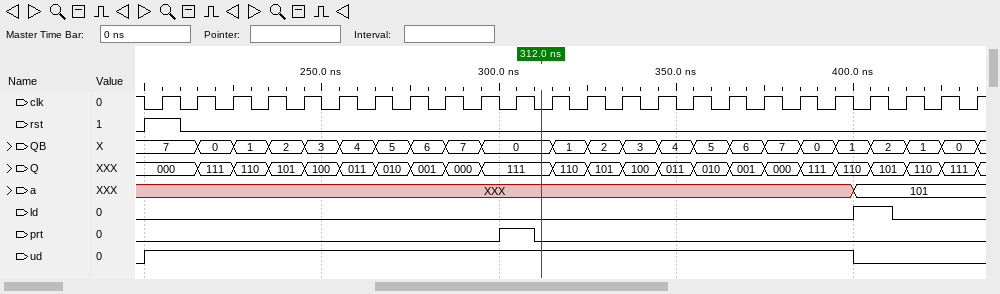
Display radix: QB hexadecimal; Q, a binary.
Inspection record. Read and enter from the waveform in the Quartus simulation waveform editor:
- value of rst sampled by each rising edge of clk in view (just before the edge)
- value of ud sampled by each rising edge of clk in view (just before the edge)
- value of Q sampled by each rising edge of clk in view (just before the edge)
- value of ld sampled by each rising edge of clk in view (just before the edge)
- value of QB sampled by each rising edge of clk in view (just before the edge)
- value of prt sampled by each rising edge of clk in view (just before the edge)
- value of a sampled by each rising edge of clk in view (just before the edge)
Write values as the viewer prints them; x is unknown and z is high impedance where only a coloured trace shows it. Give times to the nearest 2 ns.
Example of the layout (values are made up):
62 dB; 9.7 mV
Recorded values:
1 0 0 0 0 0 0 0 0 0 0 0 0 0 0 0 0 0 0 0 0 0 0 0; 1 1 1 1 1 1 1 1 1 1 1 1 1 1 1 1 1 1 1 1 0 0 0 0; 000, 000, 111, 110, 101, 100, 011, 010, 001, 000, 111, 111, 110, 101, 100, 011, 010, 001, 000, 111, 110, 101, 110, 111; 0 0 0 0 0 0 0 0 0 0 0 0 0 0 0 0 0 0 0 0 1 0 0 0; 7, 7, 0, 1, 2, 3, 4, 5, 6, 7, 0, 0, 1, 2, 3, 4, 5, 6, 7, 0, 1, 2, 1, 0; 0 0 0 0 0 0 0 0 0 0 1 0 0 0 0 0 0 0 0 0 0 0 0 0; XXX, XXX, XXX, XXX, XXX, XXX, XXX, XXX, XXX, XXX, XXX, XXX, XXX, XXX, XXX, XXX, XXX, XXX, XXX, XXX, 101, 101, 101, 101
